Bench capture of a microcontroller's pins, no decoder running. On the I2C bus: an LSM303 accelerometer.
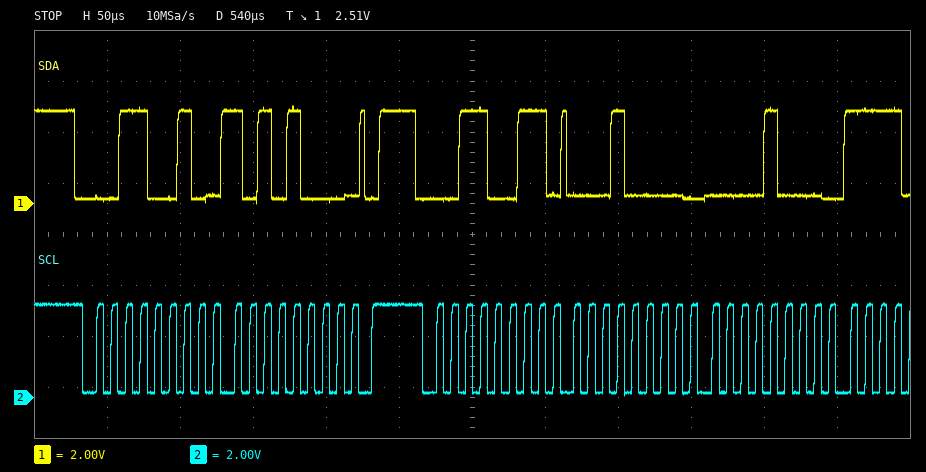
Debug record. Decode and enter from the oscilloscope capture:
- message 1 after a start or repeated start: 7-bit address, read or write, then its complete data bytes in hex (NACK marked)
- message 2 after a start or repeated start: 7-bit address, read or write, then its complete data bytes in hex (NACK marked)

0x19 write: A8
0x19 read: 10 08
